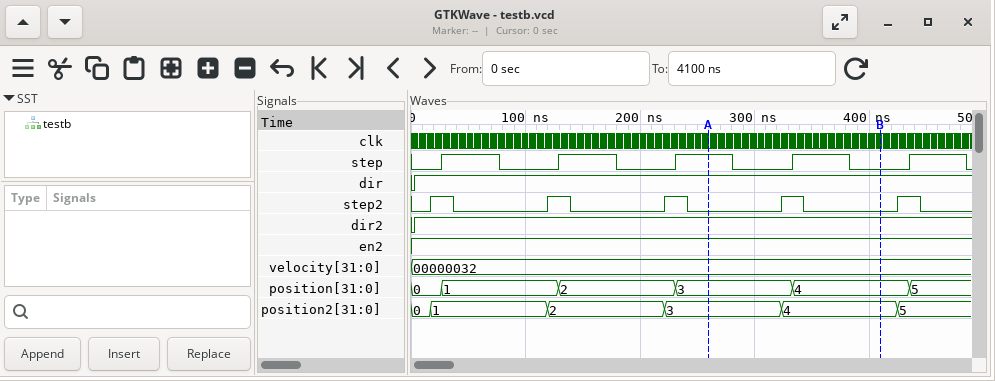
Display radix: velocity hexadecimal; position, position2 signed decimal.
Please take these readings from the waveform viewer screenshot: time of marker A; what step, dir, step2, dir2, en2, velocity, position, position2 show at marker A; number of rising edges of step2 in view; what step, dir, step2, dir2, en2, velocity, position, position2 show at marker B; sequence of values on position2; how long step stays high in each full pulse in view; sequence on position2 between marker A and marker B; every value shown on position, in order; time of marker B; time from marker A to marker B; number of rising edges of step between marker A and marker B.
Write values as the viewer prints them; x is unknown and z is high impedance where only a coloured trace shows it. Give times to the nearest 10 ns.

260 ns
step=1, dir=1, step2=0, dir2=1, en2=1, velocity=00000032, position=3, position2=3
5
step=0, dir=1, step2=0, dir2=1, en2=1, velocity=00000032, position=4, position2=4
0, 1, 2, 3, 4, 5
50 ns, 50 ns, 50 ns, 50 ns, 50 ns
3, 4
0, 1, 2, 3, 4, 5
410 ns
150 ns
1
